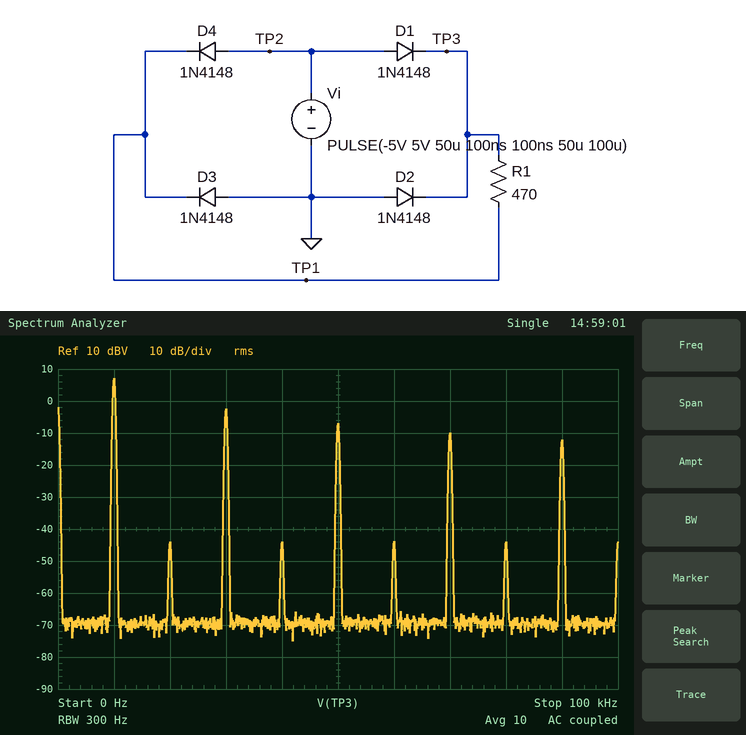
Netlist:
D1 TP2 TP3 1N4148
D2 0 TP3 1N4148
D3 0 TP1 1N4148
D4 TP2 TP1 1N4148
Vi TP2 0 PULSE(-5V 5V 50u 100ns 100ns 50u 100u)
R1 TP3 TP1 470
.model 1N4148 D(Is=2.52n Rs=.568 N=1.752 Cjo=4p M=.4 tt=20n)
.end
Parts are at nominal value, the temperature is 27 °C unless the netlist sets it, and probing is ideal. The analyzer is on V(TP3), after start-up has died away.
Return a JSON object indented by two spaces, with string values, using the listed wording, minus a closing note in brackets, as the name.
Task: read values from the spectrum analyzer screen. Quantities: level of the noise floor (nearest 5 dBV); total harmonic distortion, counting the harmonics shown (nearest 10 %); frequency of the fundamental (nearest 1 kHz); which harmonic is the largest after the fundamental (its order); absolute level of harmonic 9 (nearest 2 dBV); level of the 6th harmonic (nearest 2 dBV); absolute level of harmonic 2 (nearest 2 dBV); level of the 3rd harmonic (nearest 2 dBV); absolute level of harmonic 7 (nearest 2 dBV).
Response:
{
  "level of the noise floor": "-70 dBV",
  "total harmonic distortion, counting the harmonics shown": "40 %",
  "frequency of the fundamental": "10 kHz",
  "which harmonic is the largest after the fundamental": "3",
  "absolute level of harmonic 9": "-12 dBV",
  "level of the 6th harmonic": "-44 dBV",
  "absolute level of harmonic 2": "-44 dBV",
  "level of the 3rd harmonic": "-2 dBV",
  "absolute level of harmonic 7": "-10 dBV"
}
